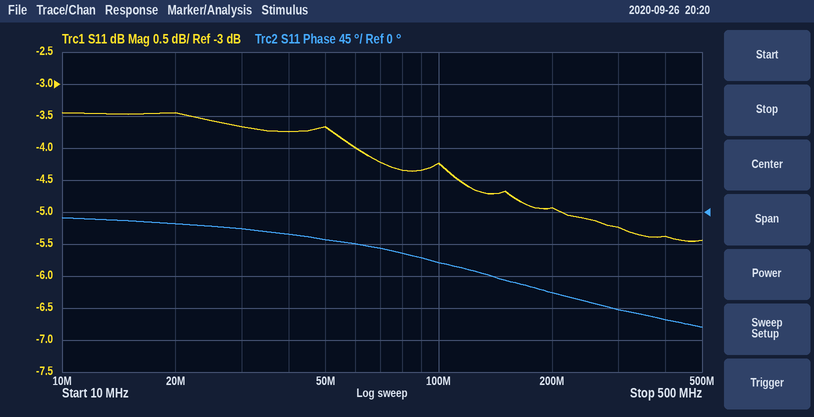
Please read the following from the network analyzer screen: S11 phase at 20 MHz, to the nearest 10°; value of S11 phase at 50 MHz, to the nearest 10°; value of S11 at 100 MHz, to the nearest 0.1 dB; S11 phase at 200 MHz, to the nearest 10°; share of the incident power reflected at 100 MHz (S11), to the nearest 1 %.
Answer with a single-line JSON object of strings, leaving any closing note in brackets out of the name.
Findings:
{"S11 phase at 20 MHz, to the nearest 10°": "-20°", "value of S11 phase at 50 MHz, to the nearest 10°": "-40°", "value of S11 at 100 MHz, to the nearest 0.1 dB": "-4.2 dB", "S11 phase at 200 MHz, to the nearest 10°": "-110°", "share of the incident power reflected at 100 MHz (S11), to the nearest 1 %": "38 %"}
